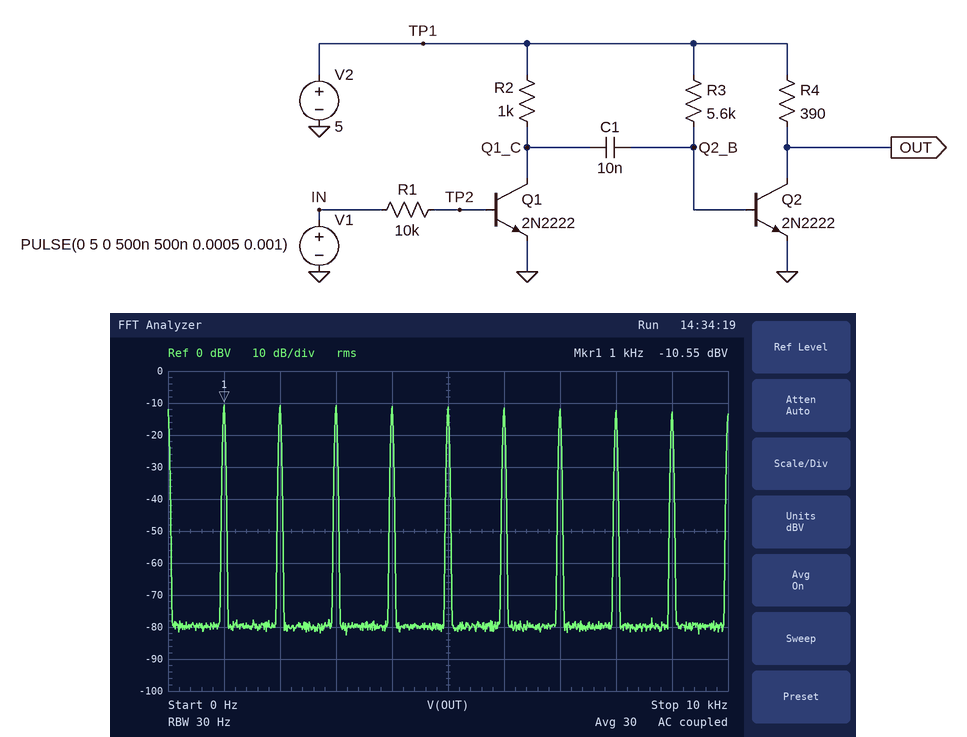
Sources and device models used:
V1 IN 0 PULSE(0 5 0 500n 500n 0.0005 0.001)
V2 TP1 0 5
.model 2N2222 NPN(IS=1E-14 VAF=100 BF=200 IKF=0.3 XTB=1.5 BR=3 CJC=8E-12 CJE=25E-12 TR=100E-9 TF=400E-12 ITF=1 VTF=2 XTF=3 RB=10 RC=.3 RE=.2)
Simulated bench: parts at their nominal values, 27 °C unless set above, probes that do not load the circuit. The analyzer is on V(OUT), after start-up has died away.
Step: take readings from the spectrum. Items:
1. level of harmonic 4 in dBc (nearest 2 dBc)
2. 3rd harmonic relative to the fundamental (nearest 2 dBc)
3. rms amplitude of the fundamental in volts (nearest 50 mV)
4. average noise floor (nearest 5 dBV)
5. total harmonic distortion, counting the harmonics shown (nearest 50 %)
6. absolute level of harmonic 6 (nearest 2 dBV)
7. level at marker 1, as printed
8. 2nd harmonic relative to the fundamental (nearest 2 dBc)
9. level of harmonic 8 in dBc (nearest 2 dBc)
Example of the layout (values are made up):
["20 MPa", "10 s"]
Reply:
["0 dBc", "0 dBc", "300 mV", "-80 dBV", "250 %", "-12 dBV", "-10.55 dBV", "0 dBc", "-2 dBc"]
